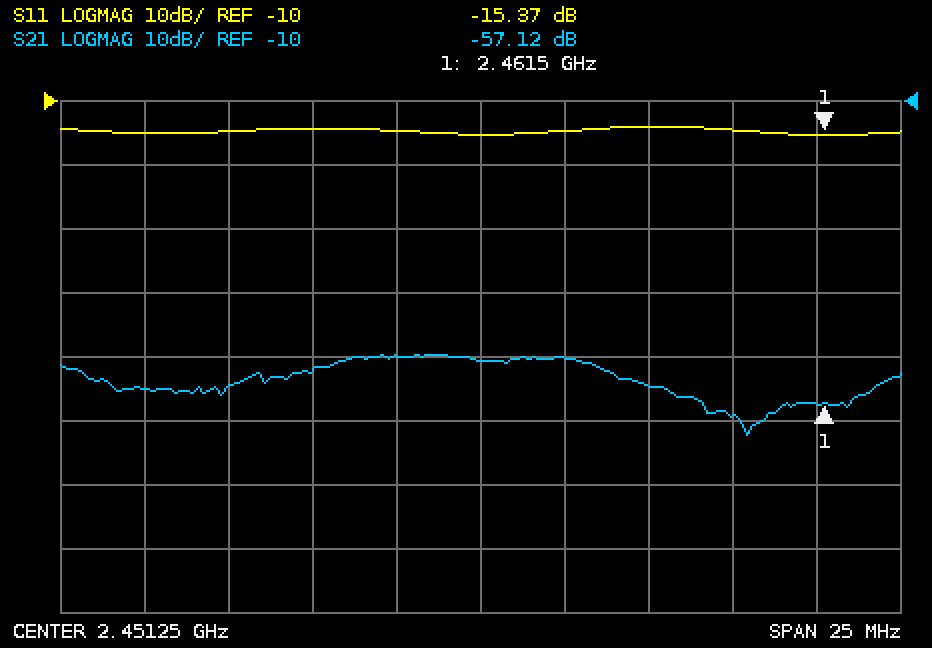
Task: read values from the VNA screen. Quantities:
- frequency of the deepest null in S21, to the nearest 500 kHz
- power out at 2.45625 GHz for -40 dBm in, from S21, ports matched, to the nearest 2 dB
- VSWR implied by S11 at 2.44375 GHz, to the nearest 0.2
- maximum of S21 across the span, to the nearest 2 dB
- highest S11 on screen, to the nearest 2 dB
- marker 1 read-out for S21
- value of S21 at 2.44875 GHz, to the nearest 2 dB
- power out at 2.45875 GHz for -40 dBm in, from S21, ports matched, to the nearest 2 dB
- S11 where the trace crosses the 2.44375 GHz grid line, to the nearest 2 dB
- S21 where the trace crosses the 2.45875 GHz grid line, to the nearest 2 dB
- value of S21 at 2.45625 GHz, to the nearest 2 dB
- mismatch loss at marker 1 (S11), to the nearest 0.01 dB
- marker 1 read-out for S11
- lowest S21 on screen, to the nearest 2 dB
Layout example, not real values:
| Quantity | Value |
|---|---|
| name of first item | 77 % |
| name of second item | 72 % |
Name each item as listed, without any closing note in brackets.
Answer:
| Quantity | Value |
|---|---|
| frequency of the deepest null in S21, to the nearest 500 kHz | 2.4590 GHz |
| power out at 2.45625 GHz for -40 dBm in, from S21, ports matched, to the nearest 2 dB | -94 dBm |
| VSWR implied by S11 at 2.44375 GHz, to the nearest 0.2 | 1.4 |
| maximum of S21 across the span, to the nearest 2 dB | -50 dB |
| highest S11 on screen, to the nearest 2 dB | -14 dB |
| marker 1 read-out for S21 | -57.12 dB |
| value of S21 at 2.44875 GHz, to the nearest 2 dB | -50 dB |
| power out at 2.45875 GHz for -40 dBm in, from S21, ports matched, to the nearest 2 dB | -100 dBm |
| S11 where the trace crosses the 2.44375 GHz grid line, to the nearest 2 dB | -14 dB |
| S21 where the trace crosses the 2.45875 GHz grid line, to the nearest 2 dB | -60 dB |
| value of S21 at 2.45625 GHz, to the nearest 2 dB | -54 dB |
| mismatch loss at marker 1 (S11), to the nearest 0.01 dB | 0.13 dB |
| marker 1 read-out for S11 | -15.37 dB |
| lowest S21 on screen, to the nearest 2 dB | -62 dB |
